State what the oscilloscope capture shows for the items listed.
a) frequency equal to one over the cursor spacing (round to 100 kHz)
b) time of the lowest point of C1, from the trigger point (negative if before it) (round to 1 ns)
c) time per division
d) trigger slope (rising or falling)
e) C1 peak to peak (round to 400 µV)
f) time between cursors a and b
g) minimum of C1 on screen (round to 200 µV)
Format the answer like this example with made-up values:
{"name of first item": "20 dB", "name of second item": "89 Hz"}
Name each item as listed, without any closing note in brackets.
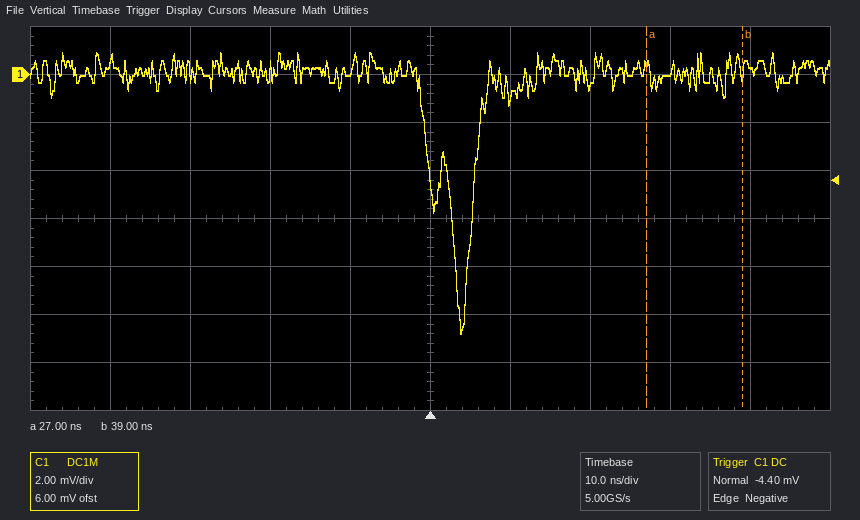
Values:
{"frequency equal to one over the cursor spacing": "83.3 MHz", "time of the lowest point of C1, from the trigger point (negative if before it)": "+4 ns", "time per division": "10 ns", "trigger slope": "falling", "C1 peak to peak": "11.6 mV", "time between cursors a and b": "12 ns", "minimum of C1 on screen": "-10.8 mV"}
